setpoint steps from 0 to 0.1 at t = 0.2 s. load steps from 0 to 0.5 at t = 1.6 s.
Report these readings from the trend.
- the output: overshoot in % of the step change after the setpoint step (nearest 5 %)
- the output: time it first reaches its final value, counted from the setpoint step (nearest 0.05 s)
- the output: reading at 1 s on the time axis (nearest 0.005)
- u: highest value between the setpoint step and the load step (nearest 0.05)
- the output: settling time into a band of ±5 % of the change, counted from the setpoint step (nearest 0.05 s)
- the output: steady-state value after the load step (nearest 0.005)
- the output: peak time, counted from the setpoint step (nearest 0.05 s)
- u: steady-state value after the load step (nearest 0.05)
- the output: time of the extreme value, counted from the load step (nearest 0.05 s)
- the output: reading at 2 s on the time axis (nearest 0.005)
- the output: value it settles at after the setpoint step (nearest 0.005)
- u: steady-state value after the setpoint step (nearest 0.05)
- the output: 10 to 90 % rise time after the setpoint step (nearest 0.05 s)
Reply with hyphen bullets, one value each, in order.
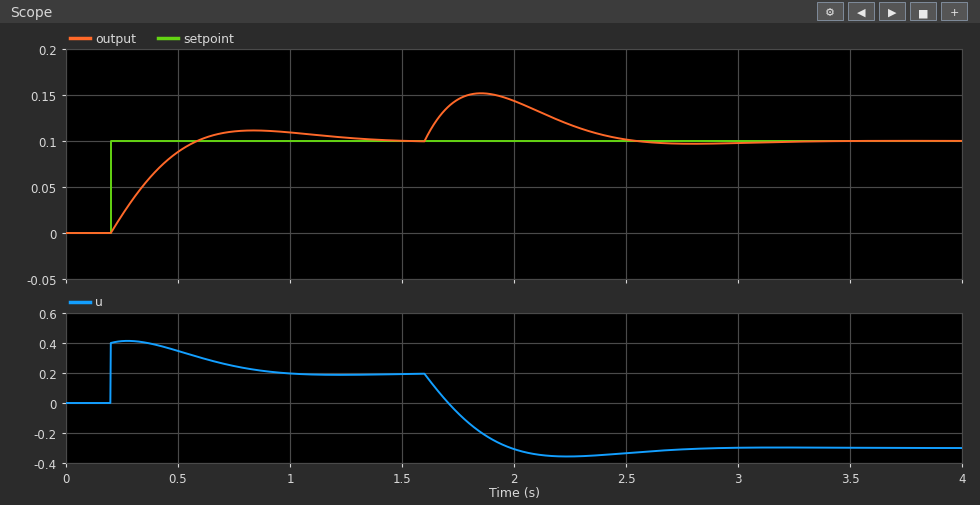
- 10 %
- 0.40 s
- 0.110
- 0.40
- 1.00 s
- 0.100
- 0.65 s
- -0.30
- 0.25 s
- 0.145
- 0.100
- 0.20
- 0.30 s
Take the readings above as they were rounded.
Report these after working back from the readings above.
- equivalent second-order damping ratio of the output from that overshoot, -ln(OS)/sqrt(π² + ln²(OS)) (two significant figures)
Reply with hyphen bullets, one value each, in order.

- 0.59
